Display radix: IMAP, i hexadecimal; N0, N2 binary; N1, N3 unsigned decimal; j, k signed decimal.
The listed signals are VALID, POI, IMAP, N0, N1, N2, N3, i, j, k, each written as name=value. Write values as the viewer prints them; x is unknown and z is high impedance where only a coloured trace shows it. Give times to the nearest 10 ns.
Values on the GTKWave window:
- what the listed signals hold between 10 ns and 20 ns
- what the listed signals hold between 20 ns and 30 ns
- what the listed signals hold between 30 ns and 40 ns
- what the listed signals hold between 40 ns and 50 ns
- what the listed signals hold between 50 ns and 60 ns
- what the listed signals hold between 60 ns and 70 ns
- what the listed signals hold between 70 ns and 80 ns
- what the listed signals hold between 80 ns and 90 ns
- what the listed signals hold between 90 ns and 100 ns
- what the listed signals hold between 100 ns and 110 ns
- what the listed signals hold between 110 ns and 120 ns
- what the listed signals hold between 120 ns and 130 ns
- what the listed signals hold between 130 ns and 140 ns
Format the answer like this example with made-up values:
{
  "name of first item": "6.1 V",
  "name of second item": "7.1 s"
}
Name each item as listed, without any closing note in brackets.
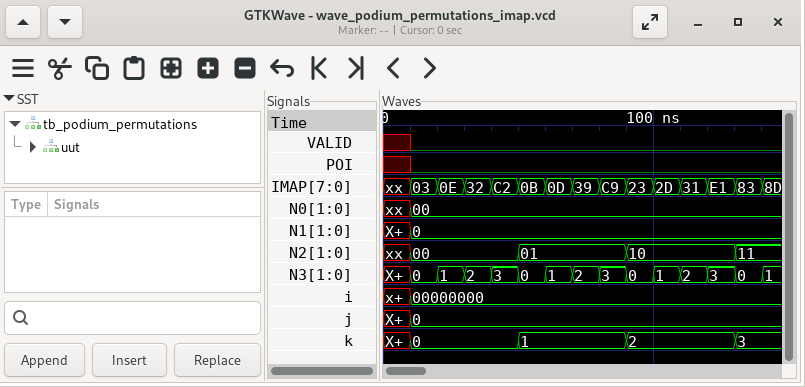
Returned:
{
  "what the listed signals hold between 10 ns and 20 ns": "VALID=0, POI=0, IMAP=03, N0=00, N1=0, N2=00, N3=0, i=00000000, j=0, k=0",
  "what the listed signals hold between 20 ns and 30 ns": "VALID=0, POI=0, IMAP=0E, N0=00, N1=0, N2=00, N3=1, i=00000000, j=0, k=0",
  "what the listed signals hold between 30 ns and 40 ns": "VALID=0, POI=0, IMAP=32, N0=00, N1=0, N2=00, N3=2, i=00000000, j=0, k=0",
  "what the listed signals hold between 40 ns and 50 ns": "VALID=0, POI=0, IMAP=C2, N0=00, N1=0, N2=00, N3=3, i=00000000, j=0, k=0",
  "what the listed signals hold between 50 ns and 60 ns": "VALID=0, POI=0, IMAP=0B, N0=00, N1=0, N2=01, N3=0, i=00000000, j=0, k=1",
  "what the listed signals hold between 60 ns and 70 ns": "VALID=0, POI=0, IMAP=0D, N0=00, N1=0, N2=01, N3=1, i=00000000, j=0, k=1",
  "what the listed signals hold between 70 ns and 80 ns": "VALID=0, POI=0, IMAP=39, N0=00, N1=0, N2=01, N3=2, i=00000000, j=0, k=1",
  "what the listed signals hold between 80 ns and 90 ns": "VALID=0, POI=0, IMAP=C9, N0=00, N1=0, N2=01, N3=3, i=00000000, j=0, k=1",
  "what the listed signals hold between 90 ns and 100 ns": "VALID=0, POI=0, IMAP=23, N0=00, N1=0, N2=10, N3=0, i=00000000, j=0, k=2",
  "what the listed signals hold between 100 ns and 110 ns": "VALID=0, POI=0, IMAP=2D, N0=00, N1=0, N2=10, N3=1, i=00000000, j=0, k=2",
  "what the listed signals hold between 110 ns and 120 ns": "VALID=0, POI=0, IMAP=31, N0=00, N1=0, N2=10, N3=2, i=00000000, j=0, k=2",
  "what the listed signals hold between 120 ns and 130 ns": "VALID=0, POI=0, IMAP=E1, N0=00, N1=0, N2=10, N3=3, i=00000000, j=0, k=2",
  "what the listed signals hold between 130 ns and 140 ns": "VALID=0, POI=0, IMAP=83, N0=00, N1=0, N2=11, N3=0, i=00000000, j=0, k=3"
}
